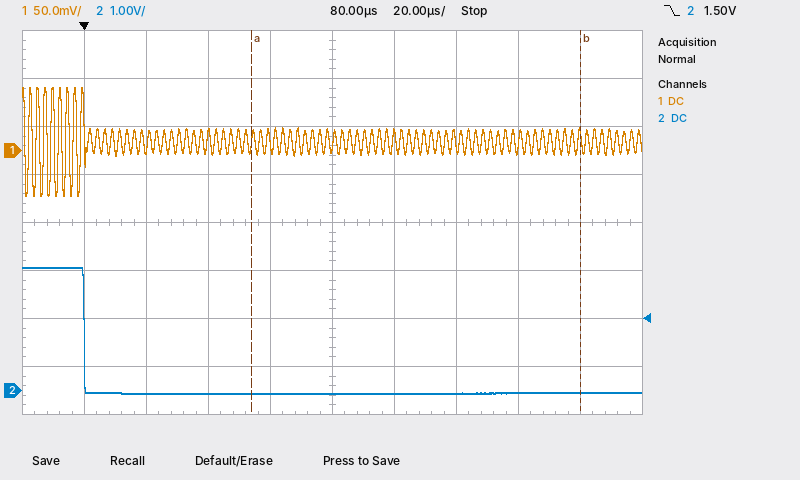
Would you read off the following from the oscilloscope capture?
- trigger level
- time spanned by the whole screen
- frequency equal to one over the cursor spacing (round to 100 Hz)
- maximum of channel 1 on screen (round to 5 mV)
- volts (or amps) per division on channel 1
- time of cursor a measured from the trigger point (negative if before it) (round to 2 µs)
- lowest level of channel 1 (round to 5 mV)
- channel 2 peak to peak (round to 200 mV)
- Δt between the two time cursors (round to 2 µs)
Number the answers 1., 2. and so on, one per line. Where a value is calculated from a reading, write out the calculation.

1. 1.50 V
2. 200 µs
3. 1 / 106 µs ≈ 9.4 kHz
4. 65 mV
5. 50 mV
6. +54 µs
7. -45 mV
8. 2.6 V
9. 106 µs
